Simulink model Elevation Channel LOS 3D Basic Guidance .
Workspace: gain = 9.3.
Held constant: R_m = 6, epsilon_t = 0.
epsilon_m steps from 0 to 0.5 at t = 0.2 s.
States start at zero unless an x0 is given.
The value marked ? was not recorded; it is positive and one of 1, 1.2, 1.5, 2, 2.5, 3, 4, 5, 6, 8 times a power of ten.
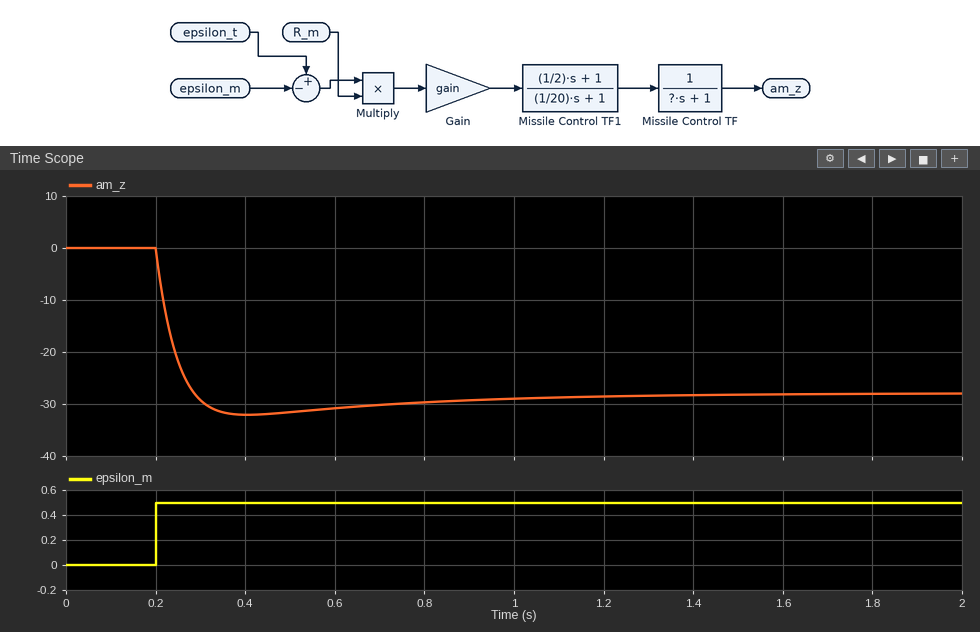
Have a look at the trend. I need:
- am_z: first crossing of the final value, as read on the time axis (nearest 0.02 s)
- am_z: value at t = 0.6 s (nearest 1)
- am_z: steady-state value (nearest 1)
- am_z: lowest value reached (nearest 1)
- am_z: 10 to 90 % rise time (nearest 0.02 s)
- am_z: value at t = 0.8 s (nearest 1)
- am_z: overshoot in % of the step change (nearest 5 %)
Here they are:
0.28 s
-31
-28
-32
0.06 s
-30
15 %
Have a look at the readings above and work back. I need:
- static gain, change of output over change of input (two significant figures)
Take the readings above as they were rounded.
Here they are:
-56
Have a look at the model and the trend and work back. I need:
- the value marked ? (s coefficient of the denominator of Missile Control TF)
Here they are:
0.4
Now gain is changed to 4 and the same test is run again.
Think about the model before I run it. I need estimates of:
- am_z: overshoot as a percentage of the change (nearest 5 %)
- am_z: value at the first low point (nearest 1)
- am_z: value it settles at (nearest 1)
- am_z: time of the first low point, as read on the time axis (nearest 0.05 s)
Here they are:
15 %
-14
-12
0.40 s
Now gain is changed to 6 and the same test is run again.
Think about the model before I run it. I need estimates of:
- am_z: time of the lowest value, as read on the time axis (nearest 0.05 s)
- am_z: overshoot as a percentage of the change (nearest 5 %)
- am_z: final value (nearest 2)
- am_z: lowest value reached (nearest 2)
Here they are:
0.40 s
15 %
-18
-20
